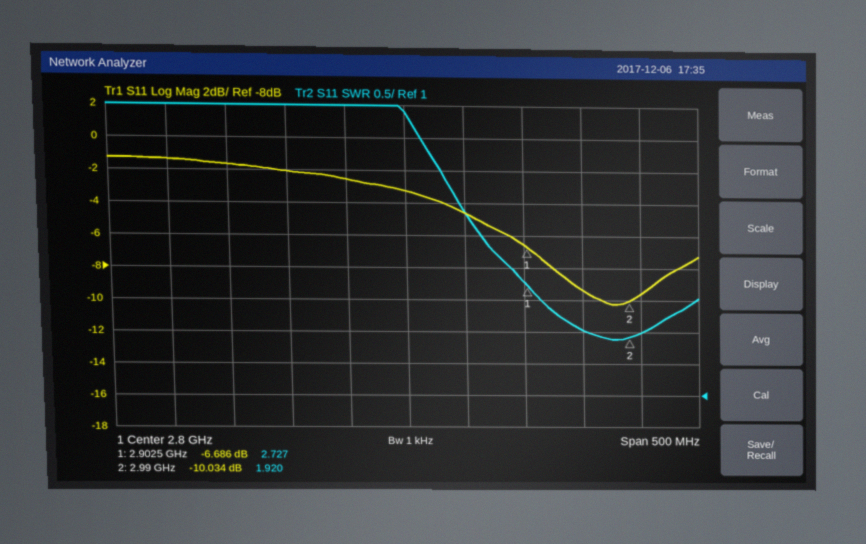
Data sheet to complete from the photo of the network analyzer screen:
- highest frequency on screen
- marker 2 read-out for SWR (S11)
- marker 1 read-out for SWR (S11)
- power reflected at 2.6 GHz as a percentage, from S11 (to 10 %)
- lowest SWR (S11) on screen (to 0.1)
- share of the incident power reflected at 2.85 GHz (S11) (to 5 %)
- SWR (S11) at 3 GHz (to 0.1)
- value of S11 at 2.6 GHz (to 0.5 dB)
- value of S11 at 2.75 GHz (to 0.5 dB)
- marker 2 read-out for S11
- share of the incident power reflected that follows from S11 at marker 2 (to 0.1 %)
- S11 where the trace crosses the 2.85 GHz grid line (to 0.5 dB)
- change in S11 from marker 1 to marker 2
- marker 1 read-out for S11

3.05 GHz
1.920
2.727
70 %
1.9
35 %
2.0
-1.5 dB
-2.5 dB
-10.034 dB
9.9 %
-4.5 dB
-3.348 dB
-6.686 dB
